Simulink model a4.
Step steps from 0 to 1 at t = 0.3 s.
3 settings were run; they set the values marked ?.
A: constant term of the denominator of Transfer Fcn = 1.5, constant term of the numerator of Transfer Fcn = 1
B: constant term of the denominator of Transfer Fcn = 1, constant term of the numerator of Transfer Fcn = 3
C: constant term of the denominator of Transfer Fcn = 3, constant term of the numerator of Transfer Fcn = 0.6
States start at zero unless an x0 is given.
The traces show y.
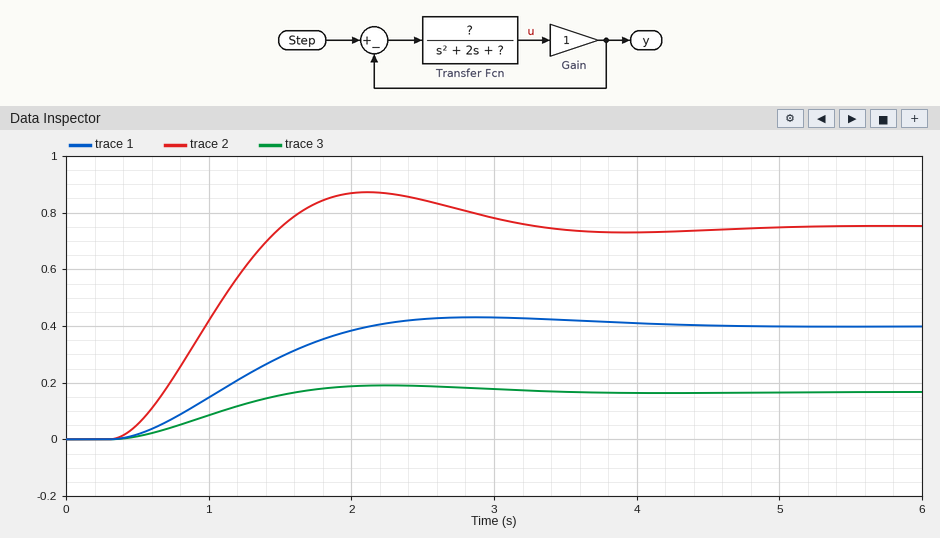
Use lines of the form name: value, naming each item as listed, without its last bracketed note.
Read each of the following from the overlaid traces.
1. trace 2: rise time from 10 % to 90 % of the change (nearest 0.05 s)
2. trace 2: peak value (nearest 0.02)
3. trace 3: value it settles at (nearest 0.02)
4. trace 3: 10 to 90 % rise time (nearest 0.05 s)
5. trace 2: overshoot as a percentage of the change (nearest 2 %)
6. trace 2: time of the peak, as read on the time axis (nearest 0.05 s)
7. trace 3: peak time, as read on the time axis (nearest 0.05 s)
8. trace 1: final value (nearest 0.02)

trace 2: rise time from 10 % to 90 % of the change: 0.80 s
trace 2: peak value: 0.88
trace 3: value it settles at: 0.16
trace 3: 10 to 90 % rise time: 0.90 s
trace 2: overshoot as a percentage of the change: 16 %
trace 2: time of the peak, as read on the time axis: 2.10 s
trace 3: peak time, as read on the time axis: 2.25 s
trace 1: final value: 0.40
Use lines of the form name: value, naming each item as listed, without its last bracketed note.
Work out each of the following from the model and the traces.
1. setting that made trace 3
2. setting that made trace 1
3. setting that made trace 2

setting that made trace 3: C
setting that made trace 1: A
setting that made trace 2: B
